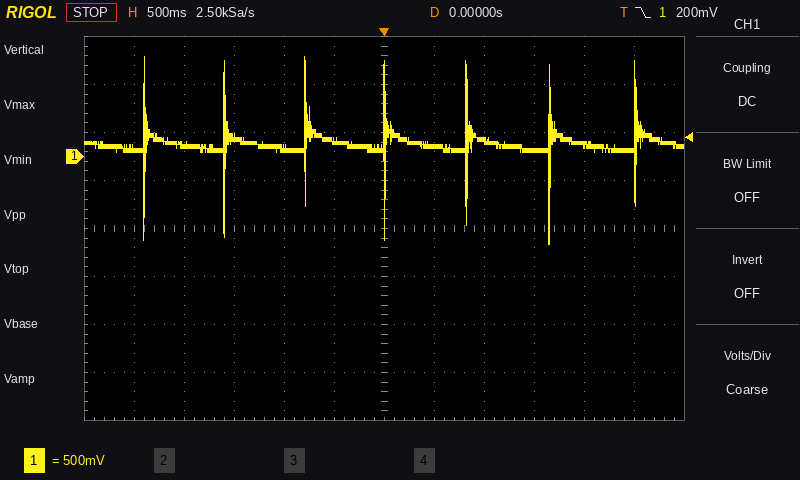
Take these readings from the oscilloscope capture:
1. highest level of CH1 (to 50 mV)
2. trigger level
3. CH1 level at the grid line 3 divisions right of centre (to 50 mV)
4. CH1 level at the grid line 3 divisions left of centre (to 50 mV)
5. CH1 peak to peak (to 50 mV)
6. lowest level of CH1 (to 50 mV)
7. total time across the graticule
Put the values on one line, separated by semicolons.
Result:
1.05 V; 200 mV; 50 mV; 200 mV; 1.95 V; -900 mV; 6 s
